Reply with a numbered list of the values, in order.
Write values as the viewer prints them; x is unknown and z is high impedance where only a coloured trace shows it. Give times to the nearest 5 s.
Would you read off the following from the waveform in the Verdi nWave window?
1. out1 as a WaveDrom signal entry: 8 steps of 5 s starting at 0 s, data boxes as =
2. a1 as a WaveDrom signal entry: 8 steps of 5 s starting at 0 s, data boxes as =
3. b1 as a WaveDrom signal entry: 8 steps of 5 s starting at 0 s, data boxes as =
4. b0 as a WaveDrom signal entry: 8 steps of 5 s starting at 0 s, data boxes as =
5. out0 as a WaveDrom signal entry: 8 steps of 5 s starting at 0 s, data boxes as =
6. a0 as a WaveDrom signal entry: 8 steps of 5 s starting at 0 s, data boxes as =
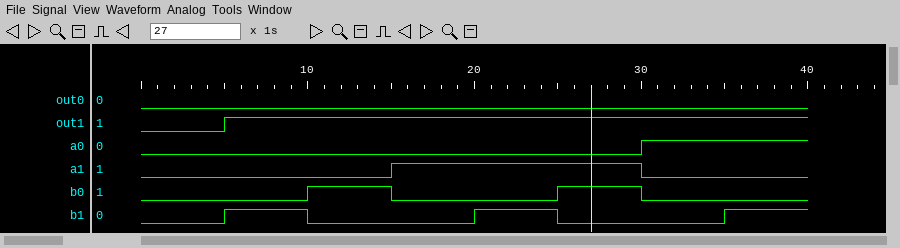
1. {name: 'out1', wave: '01......'}
2. {name: 'a1', wave: '0..1..0.'}
3. {name: 'b1', wave: '010.10.1'}
4. {name: 'b0', wave: '0.10.10.'}
5. {name: 'out0', wave: '0.......'}
6. {name: 'a0', wave: '0.....1.'}
